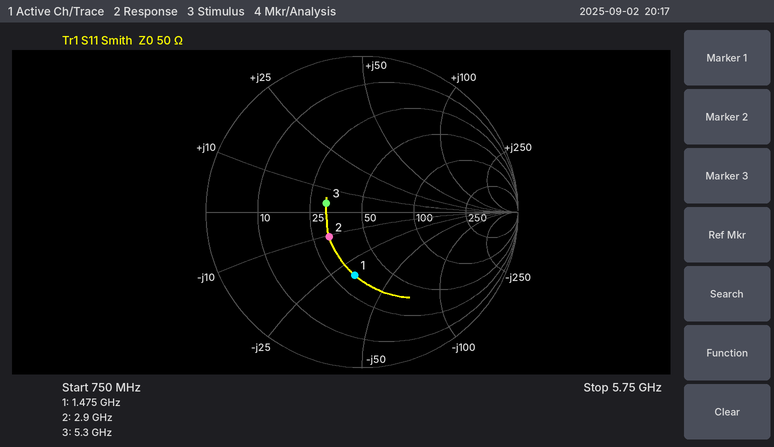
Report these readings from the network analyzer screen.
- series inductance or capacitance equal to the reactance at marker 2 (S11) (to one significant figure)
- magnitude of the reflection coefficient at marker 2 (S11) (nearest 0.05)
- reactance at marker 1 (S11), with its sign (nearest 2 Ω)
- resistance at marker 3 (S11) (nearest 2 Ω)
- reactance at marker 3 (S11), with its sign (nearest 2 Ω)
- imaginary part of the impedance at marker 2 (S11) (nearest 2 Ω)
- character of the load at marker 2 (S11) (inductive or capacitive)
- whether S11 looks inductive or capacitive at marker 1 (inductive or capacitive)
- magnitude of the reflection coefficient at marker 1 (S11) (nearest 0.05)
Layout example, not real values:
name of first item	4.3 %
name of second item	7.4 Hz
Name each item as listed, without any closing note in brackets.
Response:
series inductance or capacitance equal to the reactance at marker 2 (S11)	5 pF
magnitude of the reflection coefficient at marker 2 (S11)	0.25
reactance at marker 1 (S11), with its sign	-32 Ω
resistance at marker 3 (S11)	32 Ω
reactance at marker 3 (S11), with its sign	+4 Ω
imaginary part of the impedance at marker 2 (S11)	-10 Ω
character of the load at marker 2 (S11)	capacitive
whether S11 looks inductive or capacitive at marker 1	capacitive
magnitude of the reflection coefficient at marker 1 (S11)	0.40
